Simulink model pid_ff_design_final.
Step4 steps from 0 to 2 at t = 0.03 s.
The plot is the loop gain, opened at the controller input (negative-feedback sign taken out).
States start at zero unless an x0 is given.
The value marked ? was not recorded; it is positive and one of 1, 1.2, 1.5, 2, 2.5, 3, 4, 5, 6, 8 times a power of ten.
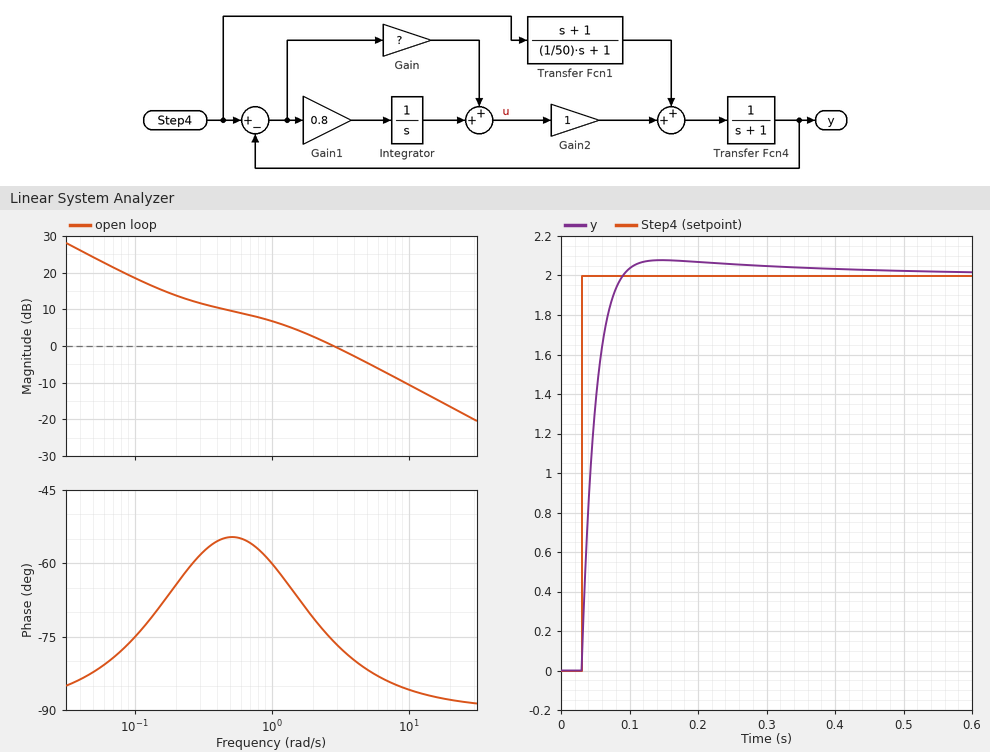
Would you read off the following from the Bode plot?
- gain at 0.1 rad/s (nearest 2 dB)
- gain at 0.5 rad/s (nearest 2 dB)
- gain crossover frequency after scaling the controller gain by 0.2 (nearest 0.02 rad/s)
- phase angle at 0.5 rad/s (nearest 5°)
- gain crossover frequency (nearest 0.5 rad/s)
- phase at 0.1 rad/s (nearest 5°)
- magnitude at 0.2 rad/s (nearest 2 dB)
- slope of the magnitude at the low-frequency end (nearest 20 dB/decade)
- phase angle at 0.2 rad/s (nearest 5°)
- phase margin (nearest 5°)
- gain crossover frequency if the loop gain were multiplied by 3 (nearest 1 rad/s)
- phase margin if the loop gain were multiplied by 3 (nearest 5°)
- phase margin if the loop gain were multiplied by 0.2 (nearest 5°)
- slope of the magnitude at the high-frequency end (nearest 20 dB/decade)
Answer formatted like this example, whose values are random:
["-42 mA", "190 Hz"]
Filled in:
["18 dB", "10 dB", "0.20 rad/s", "-55°", "3.0 rad/s", "-75°", "14 dB", "-20 dB/decade", "-65°", "105°", "9 rad/s", "95°", "115°", "-20 dB/decade"]
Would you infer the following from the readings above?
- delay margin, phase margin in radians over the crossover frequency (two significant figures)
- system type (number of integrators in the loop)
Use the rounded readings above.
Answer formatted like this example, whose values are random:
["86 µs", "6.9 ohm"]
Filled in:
["0.61 s", "1"]
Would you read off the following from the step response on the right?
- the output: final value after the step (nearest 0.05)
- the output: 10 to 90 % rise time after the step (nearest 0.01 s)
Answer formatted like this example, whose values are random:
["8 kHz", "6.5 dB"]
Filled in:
["2.00", "0.04 s"]
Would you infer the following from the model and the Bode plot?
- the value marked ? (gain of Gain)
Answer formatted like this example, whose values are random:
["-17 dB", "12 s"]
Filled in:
["3"]
